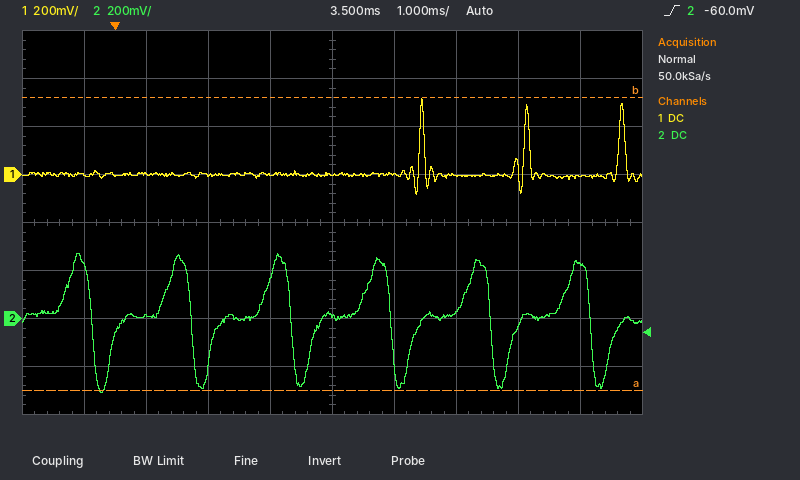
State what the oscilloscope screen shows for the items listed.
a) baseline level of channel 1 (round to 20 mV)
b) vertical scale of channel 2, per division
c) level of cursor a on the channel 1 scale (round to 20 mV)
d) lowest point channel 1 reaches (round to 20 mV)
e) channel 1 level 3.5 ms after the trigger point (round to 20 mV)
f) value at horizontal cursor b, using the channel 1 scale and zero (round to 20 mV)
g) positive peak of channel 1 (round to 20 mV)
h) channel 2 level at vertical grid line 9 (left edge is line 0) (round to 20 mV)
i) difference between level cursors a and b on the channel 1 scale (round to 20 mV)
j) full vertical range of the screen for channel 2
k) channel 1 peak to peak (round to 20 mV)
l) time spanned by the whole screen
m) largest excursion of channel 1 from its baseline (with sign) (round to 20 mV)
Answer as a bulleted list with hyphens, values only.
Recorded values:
- 0 mV
- 200 mV
- -900 mV
- -80 mV
- 0 mV
- 320 mV
- 320 mV
- 220 mV
- 1.22 V
- 1.6 V
- 400 mV
- 10 ms
- +320 mV
